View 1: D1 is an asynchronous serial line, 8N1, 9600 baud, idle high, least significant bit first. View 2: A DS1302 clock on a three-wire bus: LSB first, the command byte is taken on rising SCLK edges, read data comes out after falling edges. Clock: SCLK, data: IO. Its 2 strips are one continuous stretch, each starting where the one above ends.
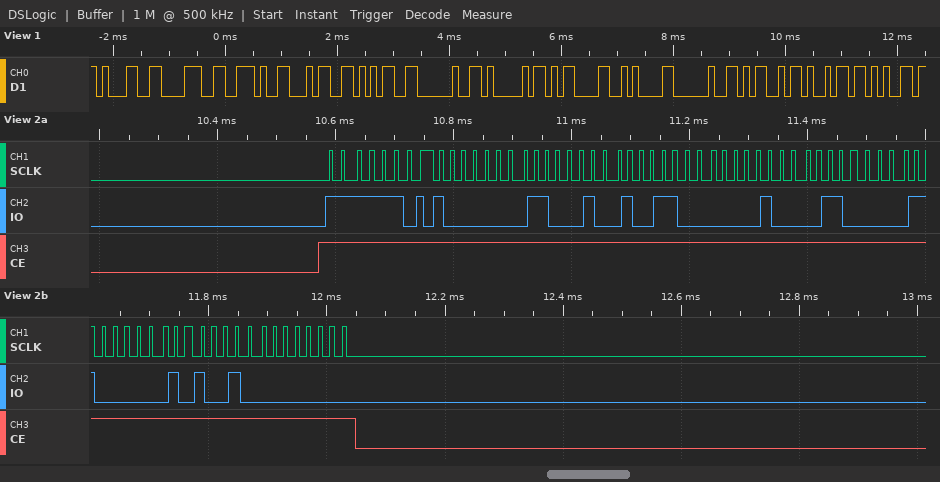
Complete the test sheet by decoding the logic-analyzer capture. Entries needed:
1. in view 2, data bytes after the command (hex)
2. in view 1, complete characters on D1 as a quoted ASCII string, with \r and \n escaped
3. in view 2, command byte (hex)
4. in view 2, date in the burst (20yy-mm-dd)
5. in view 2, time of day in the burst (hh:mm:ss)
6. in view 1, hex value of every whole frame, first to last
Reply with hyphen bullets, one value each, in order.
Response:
- 01 23 19 10 06 03 25 00
- "18.45 A\r\n Mie"
- 0xBF
- 2025-06-10
- 19:23:01
- 31 38 2E 34 35 20 41 0D 0A 20 4D 69 65
